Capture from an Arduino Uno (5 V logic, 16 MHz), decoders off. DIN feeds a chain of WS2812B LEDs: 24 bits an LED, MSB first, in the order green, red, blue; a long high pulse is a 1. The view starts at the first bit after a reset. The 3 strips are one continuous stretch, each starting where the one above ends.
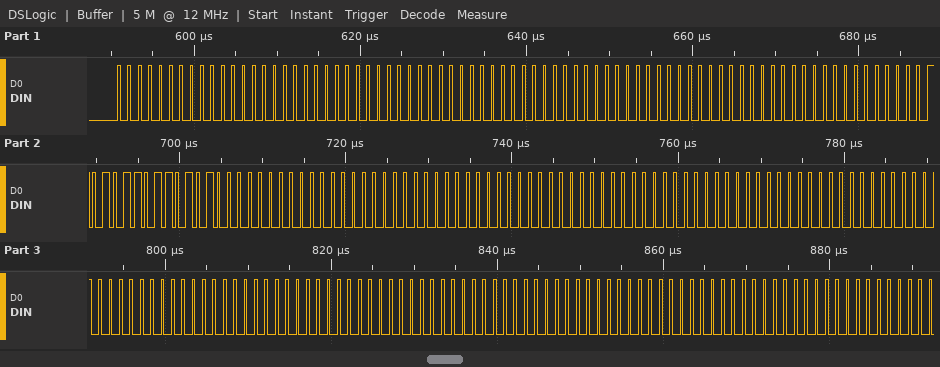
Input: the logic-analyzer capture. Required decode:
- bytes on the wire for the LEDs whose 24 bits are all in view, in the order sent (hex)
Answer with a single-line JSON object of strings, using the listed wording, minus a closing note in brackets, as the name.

{"bytes on the wire for the LEDs whose 24 bits are all in view, in the order sent": "00 00 00 00 00 00 00 00 00 02 B6 A0 00 00 00 00 00 00 00 00 00 00 00 00 00 00 00 00 00 00"}
